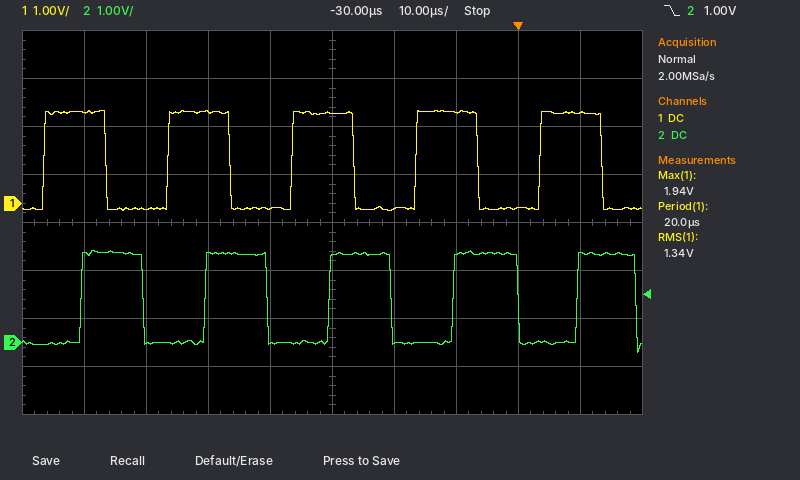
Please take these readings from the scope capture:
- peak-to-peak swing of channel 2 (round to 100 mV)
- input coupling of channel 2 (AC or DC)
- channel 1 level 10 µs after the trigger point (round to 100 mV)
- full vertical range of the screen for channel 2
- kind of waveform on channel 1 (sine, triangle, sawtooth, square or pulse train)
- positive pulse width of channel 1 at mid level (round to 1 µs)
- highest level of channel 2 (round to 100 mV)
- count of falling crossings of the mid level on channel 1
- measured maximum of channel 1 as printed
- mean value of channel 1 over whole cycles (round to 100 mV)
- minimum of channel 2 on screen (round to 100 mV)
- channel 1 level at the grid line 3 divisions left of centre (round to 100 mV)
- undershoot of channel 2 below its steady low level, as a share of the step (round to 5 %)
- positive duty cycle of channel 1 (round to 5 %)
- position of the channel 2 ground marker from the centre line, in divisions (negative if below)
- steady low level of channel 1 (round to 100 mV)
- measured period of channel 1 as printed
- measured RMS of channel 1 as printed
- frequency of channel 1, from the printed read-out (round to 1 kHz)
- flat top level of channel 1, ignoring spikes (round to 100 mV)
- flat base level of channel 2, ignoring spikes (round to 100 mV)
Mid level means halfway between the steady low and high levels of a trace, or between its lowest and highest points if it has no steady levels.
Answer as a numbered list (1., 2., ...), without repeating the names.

1. 2.1 V
2. DC
3. 1.9 V
4. 8 V
5. square
6. 10 µs
7. 1.9 V
8. 5
9. 1.94 V
10. 900 mV
11. -200 mV
12. -100 mV
13. 10 %
14. 50 %
15. -2.5 div
16. -100 mV
17. 20.0 µs
18. 1.34 V
19. 50 kHz
20. 1.9 V
21. 0.0 V
